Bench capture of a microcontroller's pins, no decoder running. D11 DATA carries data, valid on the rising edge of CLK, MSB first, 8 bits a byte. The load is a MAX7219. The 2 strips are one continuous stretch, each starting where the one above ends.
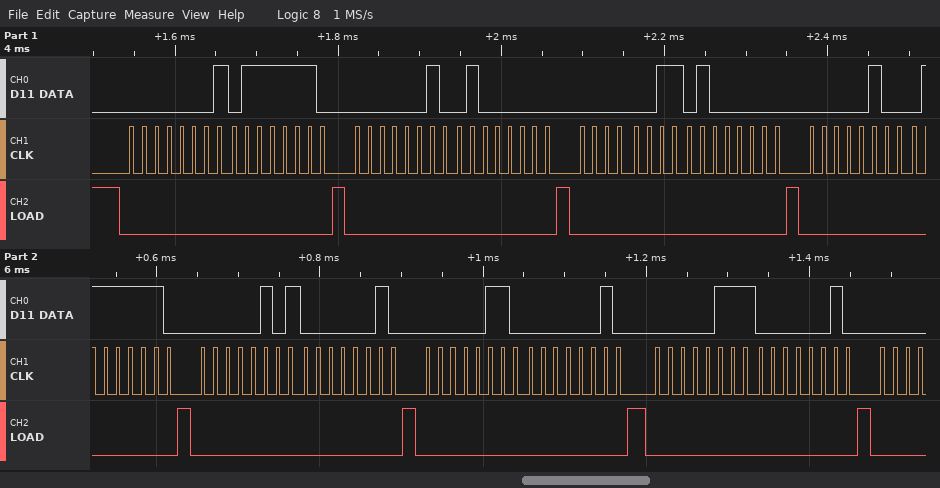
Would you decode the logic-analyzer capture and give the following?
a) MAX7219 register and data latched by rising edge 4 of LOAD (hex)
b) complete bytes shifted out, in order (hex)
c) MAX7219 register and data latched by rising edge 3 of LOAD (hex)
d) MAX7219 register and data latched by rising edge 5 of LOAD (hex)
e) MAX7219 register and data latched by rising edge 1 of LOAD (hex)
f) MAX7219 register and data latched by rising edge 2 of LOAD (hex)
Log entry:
register 0x4, data 0x7E
01 7E 02 40 03 40 04 7E 05 02 06 02 07 02
register 0x3, data 0x40
register 0x5, data 0x02
register 0x1, data 0x7E
register 0x2, data 0x40
